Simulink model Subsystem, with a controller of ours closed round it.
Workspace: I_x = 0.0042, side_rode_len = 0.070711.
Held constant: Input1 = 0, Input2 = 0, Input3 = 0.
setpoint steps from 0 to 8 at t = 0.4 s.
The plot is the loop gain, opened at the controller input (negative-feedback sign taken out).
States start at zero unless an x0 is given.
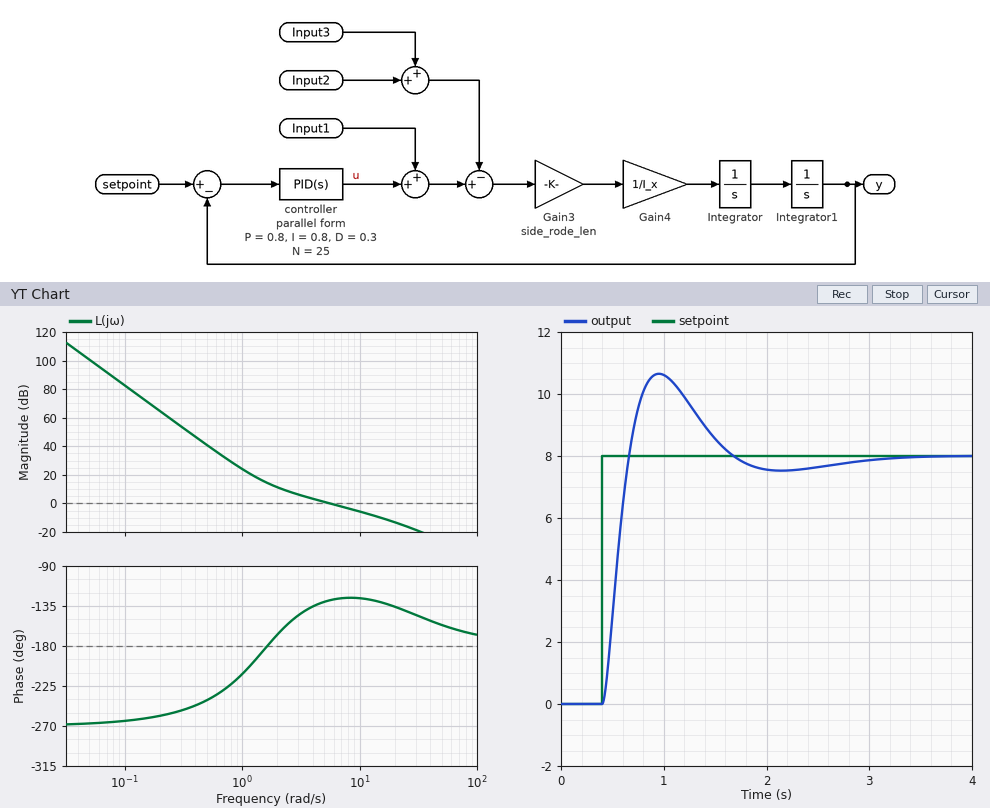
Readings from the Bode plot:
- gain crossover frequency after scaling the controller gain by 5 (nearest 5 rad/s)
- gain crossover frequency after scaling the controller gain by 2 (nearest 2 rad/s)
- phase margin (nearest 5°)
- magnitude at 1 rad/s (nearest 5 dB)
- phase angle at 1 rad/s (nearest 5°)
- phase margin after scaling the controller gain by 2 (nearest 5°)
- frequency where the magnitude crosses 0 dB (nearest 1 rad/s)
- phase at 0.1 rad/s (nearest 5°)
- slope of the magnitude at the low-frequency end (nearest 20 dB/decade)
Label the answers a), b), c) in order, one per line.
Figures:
a) 20 rad/s
b) 10 rad/s
c) 50°
d) 25 dB
e) -210°
f) 55°
g) 6 rad/s
h) -265°
i) -60 dB/decade
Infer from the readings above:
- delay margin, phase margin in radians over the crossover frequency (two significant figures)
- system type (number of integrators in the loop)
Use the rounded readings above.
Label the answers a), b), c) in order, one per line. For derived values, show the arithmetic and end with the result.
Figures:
a) 50 × π / 180 / 6 = 0.15 s
b) 3
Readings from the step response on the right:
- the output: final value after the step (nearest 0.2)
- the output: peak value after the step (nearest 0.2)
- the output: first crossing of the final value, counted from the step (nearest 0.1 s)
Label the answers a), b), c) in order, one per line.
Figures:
a) 8.0
b) 10.6
c) 0.3 s
